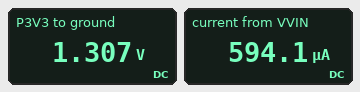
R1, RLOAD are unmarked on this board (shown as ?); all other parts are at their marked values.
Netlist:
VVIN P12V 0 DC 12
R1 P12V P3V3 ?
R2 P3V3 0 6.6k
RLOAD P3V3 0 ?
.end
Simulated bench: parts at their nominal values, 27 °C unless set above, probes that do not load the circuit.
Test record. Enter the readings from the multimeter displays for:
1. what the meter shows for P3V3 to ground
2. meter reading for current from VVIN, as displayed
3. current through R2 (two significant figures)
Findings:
1.307 V
594.1 µA
200 µA
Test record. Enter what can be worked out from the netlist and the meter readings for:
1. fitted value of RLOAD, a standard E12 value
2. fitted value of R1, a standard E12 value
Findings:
3.3 kΩ
18 kΩ
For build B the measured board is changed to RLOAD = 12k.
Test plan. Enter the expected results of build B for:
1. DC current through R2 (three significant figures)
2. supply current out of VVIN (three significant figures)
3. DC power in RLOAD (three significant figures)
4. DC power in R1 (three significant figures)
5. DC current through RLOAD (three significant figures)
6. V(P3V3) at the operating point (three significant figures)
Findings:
348 µA
539 µA
439 µW
5.23 mW
191 µA
2.30 V
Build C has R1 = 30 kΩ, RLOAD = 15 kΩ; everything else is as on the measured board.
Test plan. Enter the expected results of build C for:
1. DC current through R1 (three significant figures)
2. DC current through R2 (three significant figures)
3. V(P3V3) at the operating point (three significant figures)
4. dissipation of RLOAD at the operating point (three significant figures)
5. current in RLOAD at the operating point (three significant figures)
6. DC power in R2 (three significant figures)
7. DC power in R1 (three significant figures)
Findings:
347 µA
241 µA
1.59 V
169 µW
106 µA
383 µW
3.61 mW
